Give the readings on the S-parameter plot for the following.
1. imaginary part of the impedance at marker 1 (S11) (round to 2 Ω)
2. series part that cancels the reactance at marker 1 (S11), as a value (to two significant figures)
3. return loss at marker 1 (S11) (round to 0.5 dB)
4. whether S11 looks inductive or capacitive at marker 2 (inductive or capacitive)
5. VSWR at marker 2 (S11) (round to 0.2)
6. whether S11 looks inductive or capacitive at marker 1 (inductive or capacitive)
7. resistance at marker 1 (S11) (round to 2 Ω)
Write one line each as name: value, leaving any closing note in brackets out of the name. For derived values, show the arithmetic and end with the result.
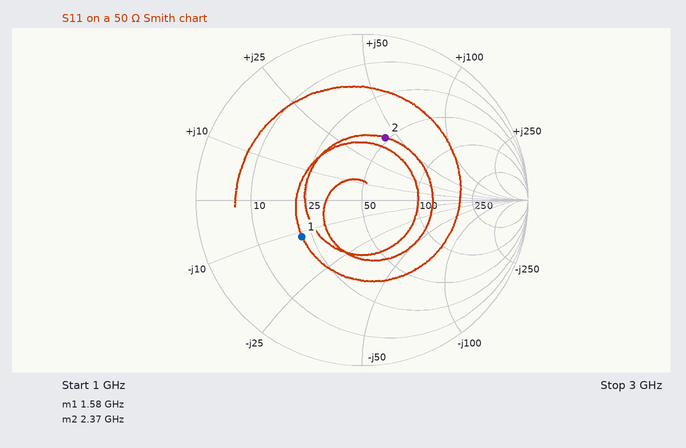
imaginary part of the impedance at marker 1 (S11): -12 Ω
series part that cancels the reactance at marker 1 (S11), as a value: L = 12 Ω/(2π × 1.58 GHz) ≈ 1.2 nH
return loss at marker 1 (S11): 7.5 dB
whether S11 looks inductive or capacitive at marker 2: inductive
VSWR at marker 2 (S11): 2.4
whether S11 looks inductive or capacitive at marker 1: capacitive
resistance at marker 1 (S11): 22 Ω
